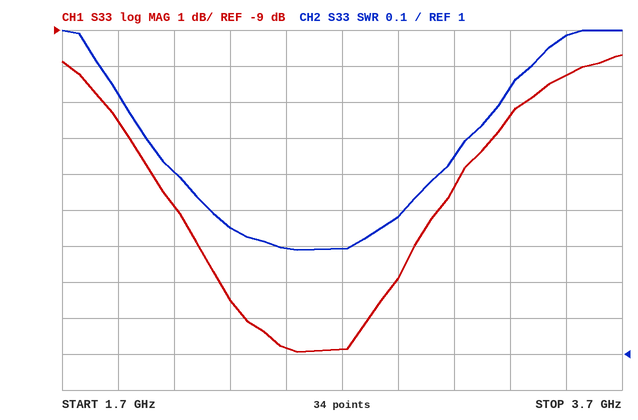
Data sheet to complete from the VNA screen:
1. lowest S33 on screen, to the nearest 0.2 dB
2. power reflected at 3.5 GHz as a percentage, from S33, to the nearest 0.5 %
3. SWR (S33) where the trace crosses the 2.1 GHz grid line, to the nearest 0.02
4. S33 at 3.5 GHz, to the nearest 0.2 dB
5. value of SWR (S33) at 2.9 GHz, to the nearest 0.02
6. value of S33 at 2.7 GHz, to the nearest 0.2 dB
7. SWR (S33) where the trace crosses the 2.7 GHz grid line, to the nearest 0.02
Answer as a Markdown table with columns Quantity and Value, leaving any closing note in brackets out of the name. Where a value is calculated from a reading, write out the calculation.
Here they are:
| Quantity | Value |
|---|---|
| lowest S33 on screen, to the nearest 0.2 dB | -18.0 dB |
| power reflected at 3.5 GHz as a percentage, from S33, to the nearest 0.5 % | 10^(-10.2/10) ≈ 9.5 % |
| SWR (S33) where the trace crosses the 2.1 GHz grid line, to the nearest 0.02 | 1.50 |
| S33 at 3.5 GHz, to the nearest 0.2 dB | -10.2 dB |
| value of SWR (S33) at 2.9 GHz, to the nearest 0.02 | 1.38 |
| value of S33 at 2.7 GHz, to the nearest 0.2 dB | -17.8 dB |
| SWR (S33) where the trace crosses the 2.7 GHz grid line, to the nearest 0.02 | 1.30 |
